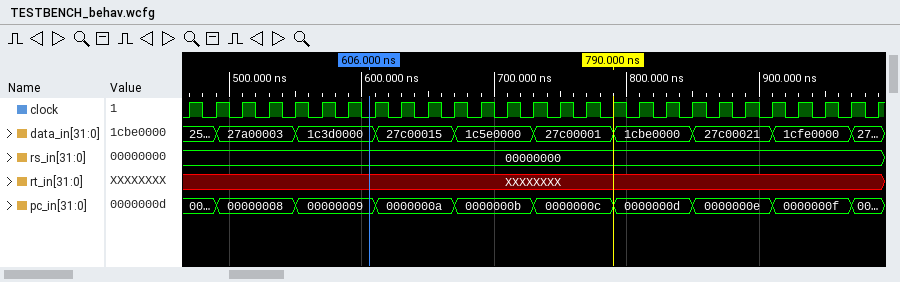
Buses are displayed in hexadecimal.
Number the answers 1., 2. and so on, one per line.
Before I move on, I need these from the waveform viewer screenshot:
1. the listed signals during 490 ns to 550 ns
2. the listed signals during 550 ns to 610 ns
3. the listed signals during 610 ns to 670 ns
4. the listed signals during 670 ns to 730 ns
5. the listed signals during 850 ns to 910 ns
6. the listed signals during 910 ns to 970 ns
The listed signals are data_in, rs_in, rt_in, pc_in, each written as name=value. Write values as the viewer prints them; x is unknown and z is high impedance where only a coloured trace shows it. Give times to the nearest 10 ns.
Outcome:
1. data_in=27a00003, rs_in=00000000, rt_in=XXXXXXXX, pc_in=00000008
2. data_in=1c3d0000, rs_in=00000000, rt_in=XXXXXXXX, pc_in=00000009
3. data_in=27c00015, rs_in=00000000, rt_in=XXXXXXXX, pc_in=0000000a
4. data_in=1c5e0000, rs_in=00000000, rt_in=XXXXXXXX, pc_in=0000000b
5. data_in=27c00021, rs_in=00000000, rt_in=XXXXXXXX, pc_in=0000000e
6. data_in=1cfe0000, rs_in=00000000, rt_in=XXXXXXXX, pc_in=0000000f
